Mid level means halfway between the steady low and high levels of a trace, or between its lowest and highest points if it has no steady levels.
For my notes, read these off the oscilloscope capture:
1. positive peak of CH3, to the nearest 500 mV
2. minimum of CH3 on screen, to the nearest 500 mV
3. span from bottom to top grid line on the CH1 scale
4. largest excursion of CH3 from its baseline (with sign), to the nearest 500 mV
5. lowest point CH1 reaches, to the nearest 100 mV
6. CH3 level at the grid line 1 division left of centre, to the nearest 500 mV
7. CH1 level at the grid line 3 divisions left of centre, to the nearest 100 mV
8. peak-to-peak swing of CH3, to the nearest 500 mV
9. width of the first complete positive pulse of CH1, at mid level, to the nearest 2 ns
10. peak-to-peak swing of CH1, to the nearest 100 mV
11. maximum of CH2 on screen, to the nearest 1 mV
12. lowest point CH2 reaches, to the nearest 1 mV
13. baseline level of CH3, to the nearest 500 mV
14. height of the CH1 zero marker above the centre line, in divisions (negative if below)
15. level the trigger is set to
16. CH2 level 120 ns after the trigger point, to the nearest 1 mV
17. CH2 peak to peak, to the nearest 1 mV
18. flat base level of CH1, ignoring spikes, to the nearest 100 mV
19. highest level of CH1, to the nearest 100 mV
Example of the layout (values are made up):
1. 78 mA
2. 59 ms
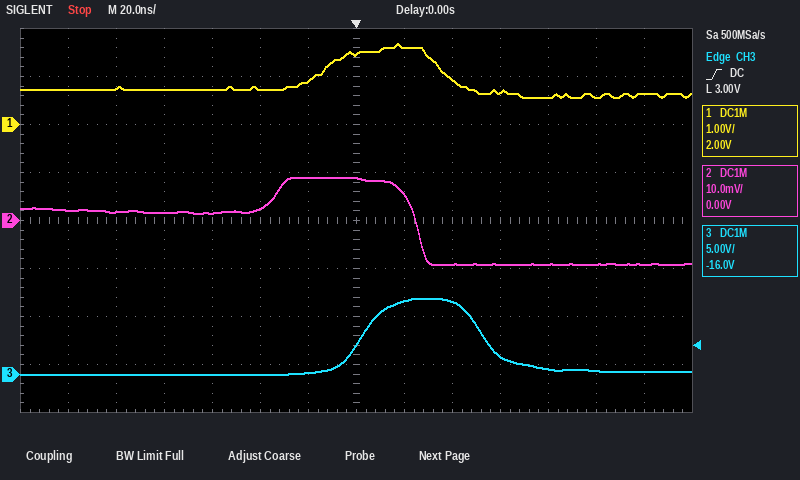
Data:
1. 8.0 V
2. 0.0 V
3. 8 V
4. +8.0 V
5. 600 mV
6. 0.0 V
7. 700 mV
8. 8.0 V
9. 48 ns
10. 1.1 V
11. 9 mV
12. -9 mV
13. 0.0 V
14. +2.0 div
15. 3.00 V
16. -9 mV
17. 18 mV
18. 700 mV
19. 1.7 V
